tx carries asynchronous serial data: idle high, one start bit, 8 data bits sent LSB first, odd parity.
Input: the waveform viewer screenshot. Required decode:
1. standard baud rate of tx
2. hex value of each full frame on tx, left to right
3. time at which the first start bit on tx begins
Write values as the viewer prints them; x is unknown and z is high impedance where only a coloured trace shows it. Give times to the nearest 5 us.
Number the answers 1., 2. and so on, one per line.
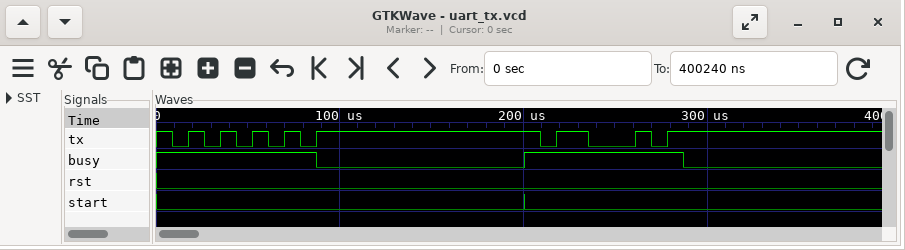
1. 115200 baud
2. 55, A3
3. 10 us
